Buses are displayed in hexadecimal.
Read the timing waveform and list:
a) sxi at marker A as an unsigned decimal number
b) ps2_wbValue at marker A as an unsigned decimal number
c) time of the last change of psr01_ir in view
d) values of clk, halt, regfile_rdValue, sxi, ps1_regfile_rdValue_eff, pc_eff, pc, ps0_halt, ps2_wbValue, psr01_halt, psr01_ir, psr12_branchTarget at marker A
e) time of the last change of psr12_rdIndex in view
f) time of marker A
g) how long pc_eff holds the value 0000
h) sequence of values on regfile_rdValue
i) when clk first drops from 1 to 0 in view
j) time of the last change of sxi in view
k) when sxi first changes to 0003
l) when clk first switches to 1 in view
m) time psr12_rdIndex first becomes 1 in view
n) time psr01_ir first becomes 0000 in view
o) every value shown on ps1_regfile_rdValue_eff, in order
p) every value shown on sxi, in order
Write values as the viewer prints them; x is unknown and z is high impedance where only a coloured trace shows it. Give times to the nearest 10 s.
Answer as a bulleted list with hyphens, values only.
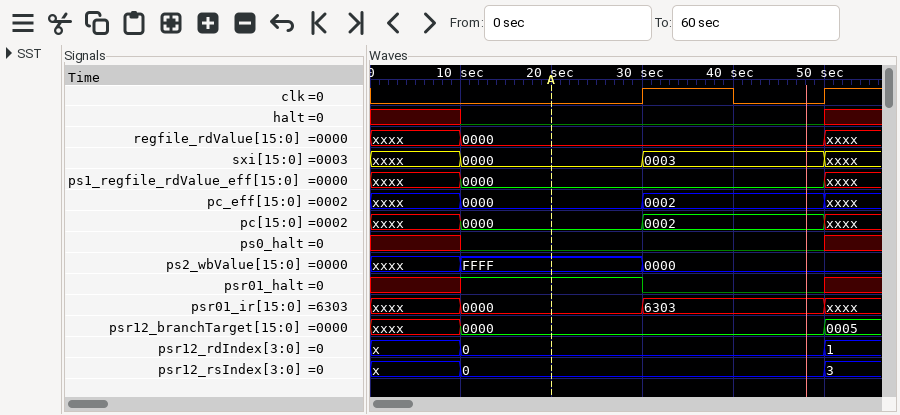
- 0
- 65535
- 50 s
- clk=0, halt=0, regfile_rdValue=0000, sxi=0000, ps1_regfile_rdValue_eff=0000, pc_eff=0000, pc=0000, ps0_halt=0, ps2_wbValue=FFFF, psr01_halt=1, psr01_ir=0000, psr12_branchTarget=0000
- 50 s
- 20 s
- 20 s
- xxxx, 0000, xxxx
- 40 s
- 50 s
- 30 s
- 30 s
- 50 s
- 10 s
- xxxx, 0000, xxxx
- xxxx, 0000, 0003, xxxx
